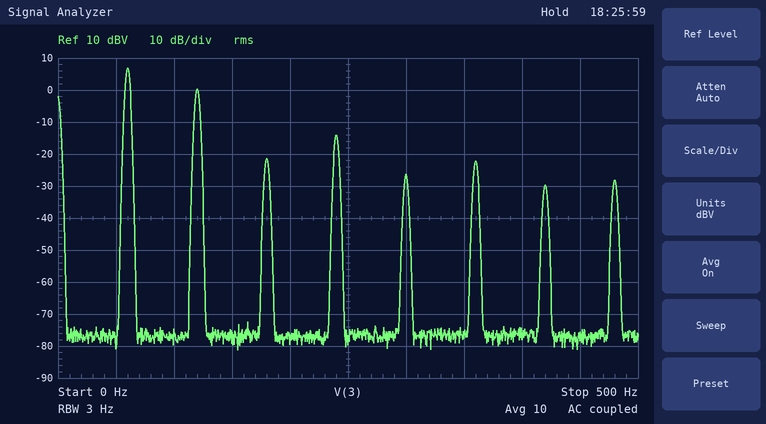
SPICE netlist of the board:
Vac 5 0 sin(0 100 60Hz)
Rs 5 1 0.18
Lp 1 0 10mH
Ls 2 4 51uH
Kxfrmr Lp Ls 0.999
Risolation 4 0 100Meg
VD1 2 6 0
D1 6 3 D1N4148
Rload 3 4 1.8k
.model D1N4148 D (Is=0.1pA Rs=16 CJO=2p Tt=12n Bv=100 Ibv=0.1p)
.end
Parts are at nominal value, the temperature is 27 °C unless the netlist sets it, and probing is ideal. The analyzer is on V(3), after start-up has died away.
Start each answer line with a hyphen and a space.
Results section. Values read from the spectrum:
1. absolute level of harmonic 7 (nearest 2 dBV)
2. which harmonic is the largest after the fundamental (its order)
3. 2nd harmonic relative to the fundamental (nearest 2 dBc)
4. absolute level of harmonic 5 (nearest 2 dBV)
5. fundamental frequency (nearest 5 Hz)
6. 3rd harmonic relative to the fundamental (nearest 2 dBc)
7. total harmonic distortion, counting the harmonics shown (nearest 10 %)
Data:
- -30 dBV
- 2
- -6 dBc
- -26 dBV
- 60 Hz
- -28 dBc
- 50 %
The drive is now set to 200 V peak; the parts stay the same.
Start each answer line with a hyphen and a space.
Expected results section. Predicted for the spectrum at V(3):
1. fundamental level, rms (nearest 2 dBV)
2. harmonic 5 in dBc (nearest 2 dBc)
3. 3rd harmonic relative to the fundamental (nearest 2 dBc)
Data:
- 14 dBV
- -40 dBc
- -34 dBc
